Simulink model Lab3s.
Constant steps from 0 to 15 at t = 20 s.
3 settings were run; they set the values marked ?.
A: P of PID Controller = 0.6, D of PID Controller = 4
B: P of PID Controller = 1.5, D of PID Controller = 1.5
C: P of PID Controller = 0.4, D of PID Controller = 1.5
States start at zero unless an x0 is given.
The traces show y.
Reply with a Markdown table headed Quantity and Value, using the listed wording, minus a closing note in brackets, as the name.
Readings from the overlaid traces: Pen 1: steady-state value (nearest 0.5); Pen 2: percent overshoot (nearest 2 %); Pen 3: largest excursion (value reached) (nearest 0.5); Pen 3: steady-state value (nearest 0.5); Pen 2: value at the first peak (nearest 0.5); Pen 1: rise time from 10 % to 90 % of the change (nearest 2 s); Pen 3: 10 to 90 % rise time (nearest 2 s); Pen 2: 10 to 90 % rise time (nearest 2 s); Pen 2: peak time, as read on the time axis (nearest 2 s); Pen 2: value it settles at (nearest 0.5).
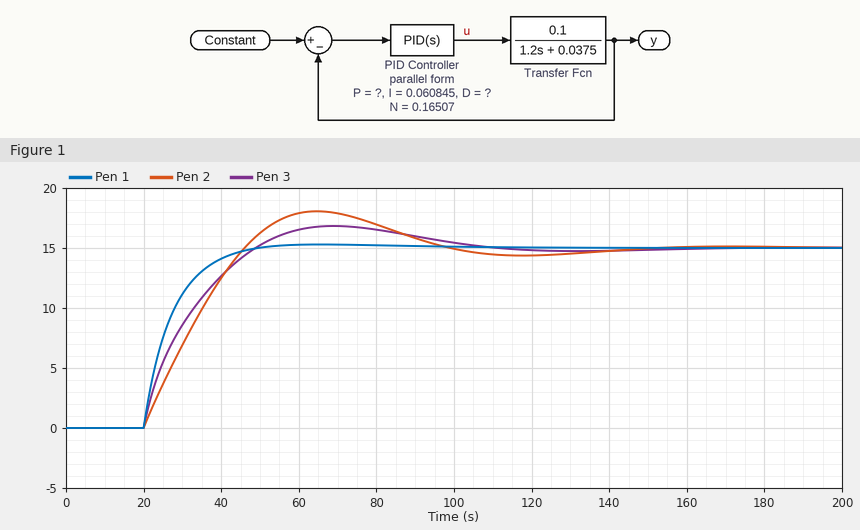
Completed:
| Quantity | Value |
|---|---|
| Pen 1: steady-state value | 15.0 |
| Pen 2: percent overshoot | 20 % |
| Pen 3: largest excursion (value reached) | 17.0 |
| Pen 3: steady-state value | 15.0 |
| Pen 2: value at the first peak | 18.0 |
| Pen 1: rise time from 10 % to 90 % of the change | 16 s |
| Pen 3: 10 to 90 % rise time | 22 s |
| Pen 2: 10 to 90 % rise time | 20 s |
| Pen 2: peak time, as read on the time axis | 64 s |
| Pen 2: value it settles at | 15.0 |
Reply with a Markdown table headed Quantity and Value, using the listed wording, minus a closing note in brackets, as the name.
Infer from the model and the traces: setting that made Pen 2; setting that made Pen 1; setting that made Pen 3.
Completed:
| Quantity | Value |
|---|---|
| setting that made Pen 2 | C |
| setting that made Pen 1 | B |
| setting that made Pen 3 | A |
